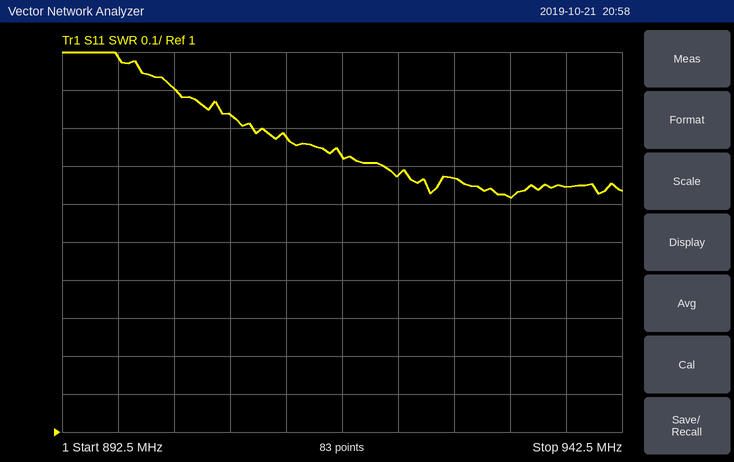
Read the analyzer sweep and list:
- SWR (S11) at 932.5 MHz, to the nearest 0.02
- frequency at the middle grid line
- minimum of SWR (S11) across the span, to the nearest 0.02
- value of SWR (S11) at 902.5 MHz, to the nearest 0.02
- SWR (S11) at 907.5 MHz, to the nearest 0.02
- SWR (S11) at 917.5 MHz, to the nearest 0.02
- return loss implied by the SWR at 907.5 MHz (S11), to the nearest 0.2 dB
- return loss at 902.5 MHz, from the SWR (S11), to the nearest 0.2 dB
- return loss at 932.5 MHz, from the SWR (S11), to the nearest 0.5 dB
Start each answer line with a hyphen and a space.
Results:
- 1.62
- 917.5 MHz
- 1.62
- 1.90
- 1.84
- 1.72
- 10.6 dB
- 10.2 dB
- 12.5 dB
